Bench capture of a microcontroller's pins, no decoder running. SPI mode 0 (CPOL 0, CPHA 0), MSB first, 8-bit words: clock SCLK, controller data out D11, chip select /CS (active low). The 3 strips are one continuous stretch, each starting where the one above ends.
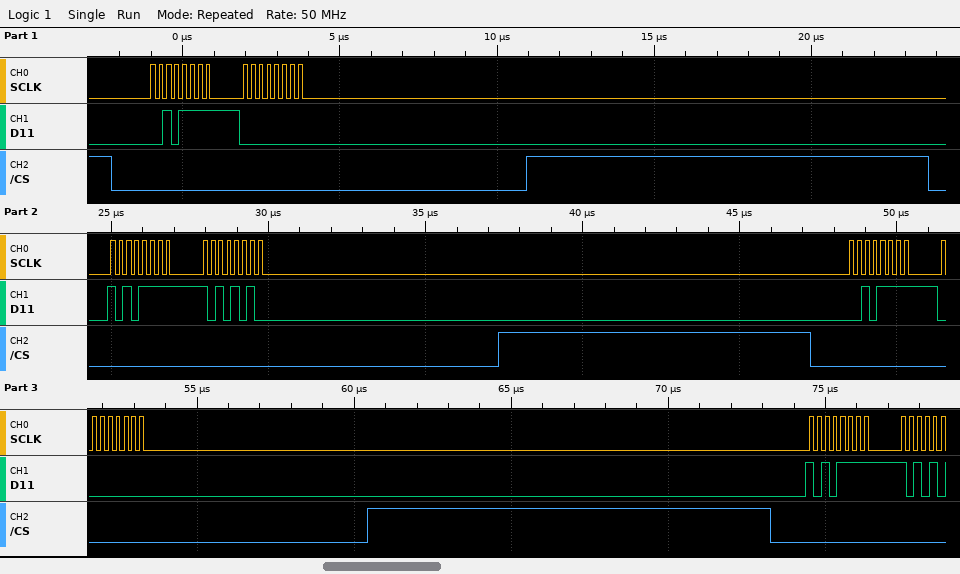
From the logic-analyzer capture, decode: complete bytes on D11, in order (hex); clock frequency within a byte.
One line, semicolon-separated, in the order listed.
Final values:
0x2F 0x00 0xAF 0xAA 0x2F 0x00 0xAF; 4 MHz
